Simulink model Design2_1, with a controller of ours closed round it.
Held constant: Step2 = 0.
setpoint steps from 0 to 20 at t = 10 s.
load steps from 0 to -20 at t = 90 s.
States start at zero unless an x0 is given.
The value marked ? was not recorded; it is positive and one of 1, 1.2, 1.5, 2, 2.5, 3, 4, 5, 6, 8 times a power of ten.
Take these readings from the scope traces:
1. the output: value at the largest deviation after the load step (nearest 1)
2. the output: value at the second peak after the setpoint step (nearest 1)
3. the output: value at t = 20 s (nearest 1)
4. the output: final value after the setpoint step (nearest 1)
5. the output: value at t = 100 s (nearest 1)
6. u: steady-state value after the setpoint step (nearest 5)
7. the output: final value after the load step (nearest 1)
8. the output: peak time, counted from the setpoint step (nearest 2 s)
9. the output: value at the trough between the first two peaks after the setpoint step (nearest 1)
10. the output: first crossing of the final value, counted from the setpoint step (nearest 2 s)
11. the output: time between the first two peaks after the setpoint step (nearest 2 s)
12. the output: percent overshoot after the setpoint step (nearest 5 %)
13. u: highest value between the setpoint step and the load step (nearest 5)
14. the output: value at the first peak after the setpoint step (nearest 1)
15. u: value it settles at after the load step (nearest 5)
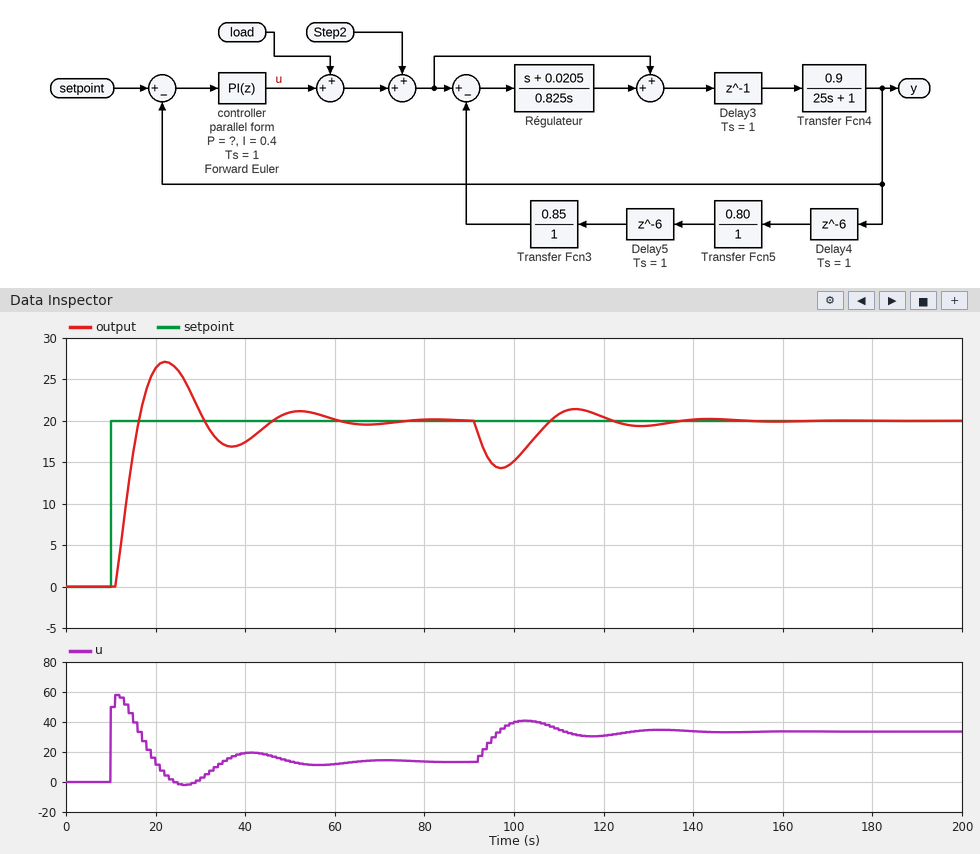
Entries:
14
21
26
20
15
15
20
12 s
17
6 s
30 s
35 %
60
27
35
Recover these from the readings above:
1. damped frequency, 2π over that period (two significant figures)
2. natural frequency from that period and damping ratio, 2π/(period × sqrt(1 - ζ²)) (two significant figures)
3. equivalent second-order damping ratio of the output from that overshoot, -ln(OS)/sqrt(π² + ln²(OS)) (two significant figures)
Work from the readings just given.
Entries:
0.21 rad/s
0.22 rad/s
0.32
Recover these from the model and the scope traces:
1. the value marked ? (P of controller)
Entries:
2.5
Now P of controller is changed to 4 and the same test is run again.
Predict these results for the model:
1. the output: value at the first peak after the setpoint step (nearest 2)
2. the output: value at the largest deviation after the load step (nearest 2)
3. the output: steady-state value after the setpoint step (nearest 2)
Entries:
24
16
20
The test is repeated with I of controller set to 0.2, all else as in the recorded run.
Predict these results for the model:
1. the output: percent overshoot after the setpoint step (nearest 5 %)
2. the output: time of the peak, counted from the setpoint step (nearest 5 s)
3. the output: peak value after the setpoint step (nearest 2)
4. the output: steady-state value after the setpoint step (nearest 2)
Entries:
15 %
15 s
24
20
